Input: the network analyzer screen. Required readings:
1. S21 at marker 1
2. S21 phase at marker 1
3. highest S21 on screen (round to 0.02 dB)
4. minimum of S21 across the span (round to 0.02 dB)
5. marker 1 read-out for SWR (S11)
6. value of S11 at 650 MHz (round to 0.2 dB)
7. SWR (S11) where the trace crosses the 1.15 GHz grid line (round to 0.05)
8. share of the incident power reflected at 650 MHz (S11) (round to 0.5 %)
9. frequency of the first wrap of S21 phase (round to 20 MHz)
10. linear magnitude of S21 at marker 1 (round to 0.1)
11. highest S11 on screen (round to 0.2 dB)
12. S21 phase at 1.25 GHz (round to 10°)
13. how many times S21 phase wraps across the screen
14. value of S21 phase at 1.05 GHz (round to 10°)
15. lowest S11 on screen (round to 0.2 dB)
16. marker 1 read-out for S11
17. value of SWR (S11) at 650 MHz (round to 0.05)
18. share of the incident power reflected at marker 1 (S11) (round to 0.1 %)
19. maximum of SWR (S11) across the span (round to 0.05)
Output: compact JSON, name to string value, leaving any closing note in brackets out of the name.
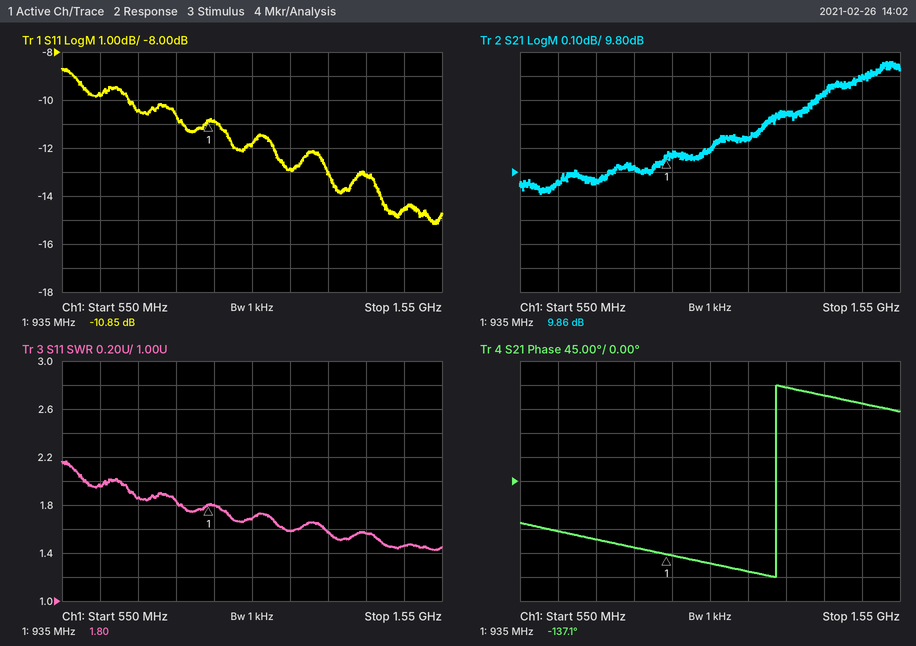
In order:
{"S21 at marker 1": "9.86 dB", "S21 phase at marker 1": "-137.1°", "highest S21 on screen": "10.26 dB", "minimum of S21 across the span": "9.70 dB", "marker 1 read-out for SWR": "1.80", "value of S11 at 650 MHz": "-9.8 dB", "SWR (S11) where the trace crosses the 1.15 GHz grid line": "1.60", "share of the incident power reflected at 650 MHz (S11)": "10.5 %", "frequency of the first wrap of S21 phase": "1.22 GHz", "linear magnitude of S21 at marker 1": "3.1", "highest S11 on screen": "-8.6 dB", "S21 phase at 1.25 GHz": "180°", "how many times S21 phase wraps across the screen": "1", "value of S21 phase at 1.05 GHz": "-150°", "lowest S11 on screen": "-15.2 dB", "marker 1 read-out for S11": "-10.85 dB", "value of SWR (S11) at 650 MHz": "1.95", "share of the incident power reflected at marker 1 (S11)": "8.2 %", "maximum of SWR (S11) across the span": "2.15"}
